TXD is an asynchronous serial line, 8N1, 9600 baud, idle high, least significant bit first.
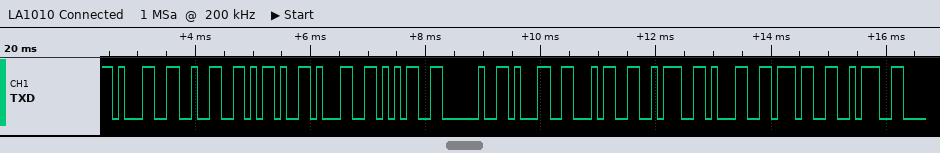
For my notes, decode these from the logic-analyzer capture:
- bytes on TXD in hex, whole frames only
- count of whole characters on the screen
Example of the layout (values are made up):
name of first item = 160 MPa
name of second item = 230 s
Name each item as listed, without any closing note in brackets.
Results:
bytes on TXD in hex, whole frames only = 0x31 0x32 0x2D 0x31 0x35 0x20 0x31 0x34 0x3A 0x31 0x37 0x3A
count of whole characters on the screen = 12
